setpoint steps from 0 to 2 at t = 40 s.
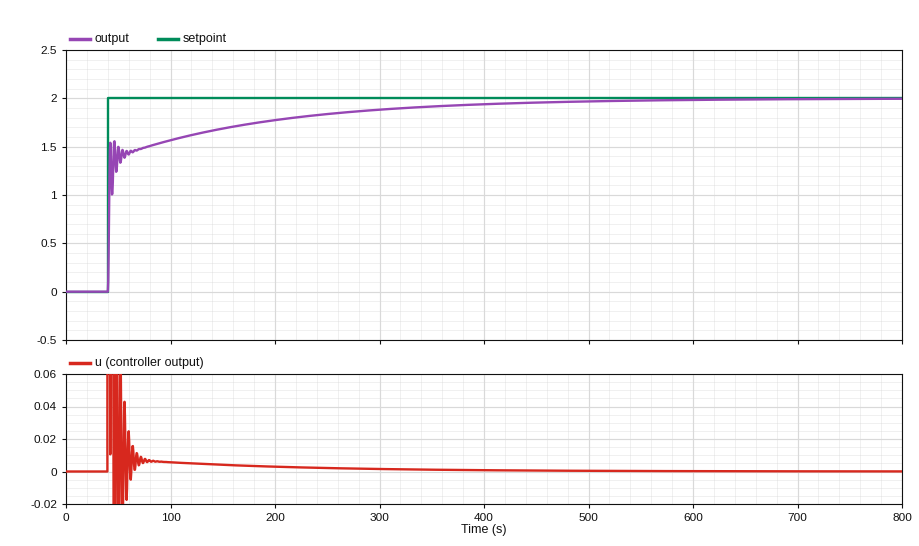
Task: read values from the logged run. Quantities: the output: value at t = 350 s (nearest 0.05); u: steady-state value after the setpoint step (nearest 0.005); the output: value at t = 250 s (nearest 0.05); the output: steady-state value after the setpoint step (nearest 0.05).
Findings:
1.90
0.000
1.85
2.00
